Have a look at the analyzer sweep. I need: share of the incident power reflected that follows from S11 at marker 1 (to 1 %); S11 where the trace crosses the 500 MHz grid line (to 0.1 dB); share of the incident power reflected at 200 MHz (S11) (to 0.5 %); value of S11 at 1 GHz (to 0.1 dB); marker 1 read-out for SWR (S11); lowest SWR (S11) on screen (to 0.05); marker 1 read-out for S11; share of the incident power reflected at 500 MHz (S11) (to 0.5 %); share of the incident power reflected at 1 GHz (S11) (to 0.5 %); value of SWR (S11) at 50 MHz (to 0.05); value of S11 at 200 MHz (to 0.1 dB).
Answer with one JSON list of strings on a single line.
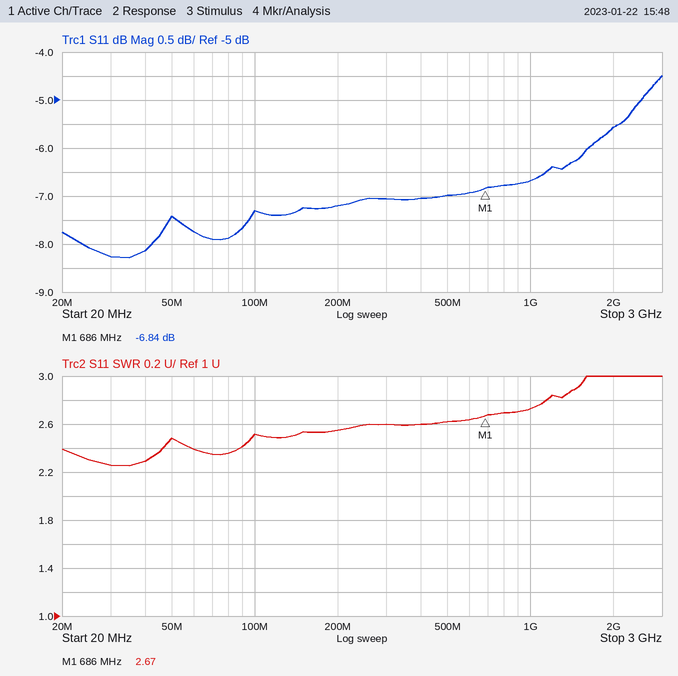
["21 %", "-7.0 dB", "19.0 %", "-6.7 dB", "2.67", "2.25", "-6.84 dB", "20.0 %", "21.5 %", "2.50", "-7.2 dB"]
